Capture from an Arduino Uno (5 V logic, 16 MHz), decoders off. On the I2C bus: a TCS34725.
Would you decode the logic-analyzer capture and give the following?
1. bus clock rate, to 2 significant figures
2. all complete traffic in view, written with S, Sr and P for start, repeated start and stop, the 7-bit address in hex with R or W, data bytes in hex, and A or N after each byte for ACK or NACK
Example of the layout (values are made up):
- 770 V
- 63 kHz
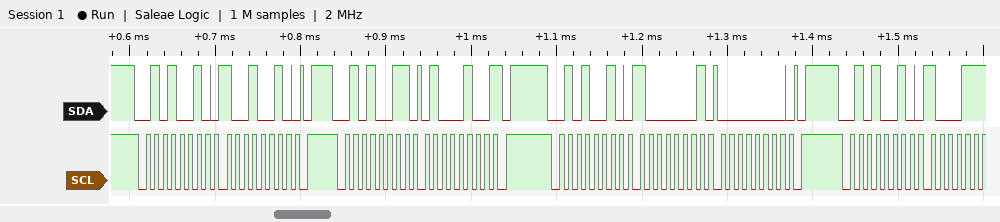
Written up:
- 100 kHz
- S 29W A 92 A P S 29R A 44 N P S 29W A 81 A 00 A P S 29W A
